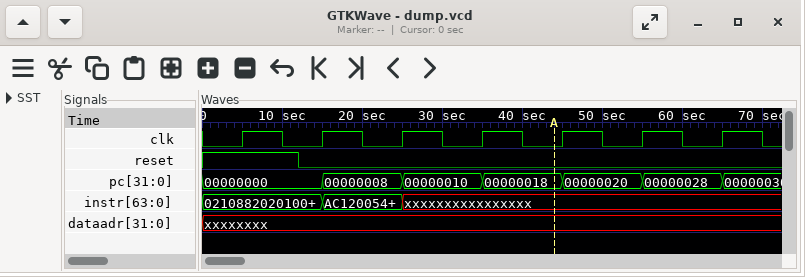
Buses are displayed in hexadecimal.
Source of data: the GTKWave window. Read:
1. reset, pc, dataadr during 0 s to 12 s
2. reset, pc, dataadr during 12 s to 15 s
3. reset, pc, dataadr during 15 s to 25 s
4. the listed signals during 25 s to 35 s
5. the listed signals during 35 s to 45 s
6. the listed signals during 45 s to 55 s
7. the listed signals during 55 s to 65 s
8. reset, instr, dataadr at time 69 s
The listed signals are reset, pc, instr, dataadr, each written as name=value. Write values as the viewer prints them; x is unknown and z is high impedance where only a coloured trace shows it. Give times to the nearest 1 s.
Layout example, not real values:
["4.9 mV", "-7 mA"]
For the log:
["reset=1, pc=00000000, dataadr=xxxxxxxx", "reset=0, pc=00000000, dataadr=xxxxxxxx", "reset=0, pc=00000008, dataadr=xxxxxxxx", "reset=0, pc=00000010, instr=xxxxxxxxxxxxxxxx, dataadr=xxxxxxxx", "reset=0, pc=00000018, instr=xxxxxxxxxxxxxxxx, dataadr=xxxxxxxx", "reset=0, pc=00000020, instr=xxxxxxxxxxxxxxxx, dataadr=xxxxxxxx", "reset=0, pc=00000028, instr=xxxxxxxxxxxxxxxx, dataadr=xxxxxxxx", "reset=0, instr=xxxxxxxxxxxxxxxx, dataadr=xxxxxxxx"]
